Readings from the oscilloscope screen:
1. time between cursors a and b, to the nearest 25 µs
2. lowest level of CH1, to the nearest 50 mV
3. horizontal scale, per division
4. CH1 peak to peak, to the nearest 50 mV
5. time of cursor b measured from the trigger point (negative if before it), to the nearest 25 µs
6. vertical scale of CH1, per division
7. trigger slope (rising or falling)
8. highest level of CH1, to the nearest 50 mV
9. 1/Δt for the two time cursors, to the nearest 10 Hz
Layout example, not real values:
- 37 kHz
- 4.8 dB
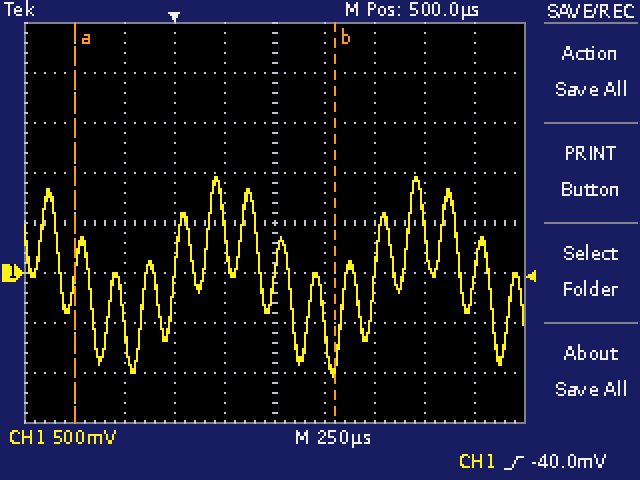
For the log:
- 1.300 ms
- -1.05 V
- 250 µs
- 2.00 V
- +800 µs
- 500 mV
- rising
- 950 mV
- 770 Hz
